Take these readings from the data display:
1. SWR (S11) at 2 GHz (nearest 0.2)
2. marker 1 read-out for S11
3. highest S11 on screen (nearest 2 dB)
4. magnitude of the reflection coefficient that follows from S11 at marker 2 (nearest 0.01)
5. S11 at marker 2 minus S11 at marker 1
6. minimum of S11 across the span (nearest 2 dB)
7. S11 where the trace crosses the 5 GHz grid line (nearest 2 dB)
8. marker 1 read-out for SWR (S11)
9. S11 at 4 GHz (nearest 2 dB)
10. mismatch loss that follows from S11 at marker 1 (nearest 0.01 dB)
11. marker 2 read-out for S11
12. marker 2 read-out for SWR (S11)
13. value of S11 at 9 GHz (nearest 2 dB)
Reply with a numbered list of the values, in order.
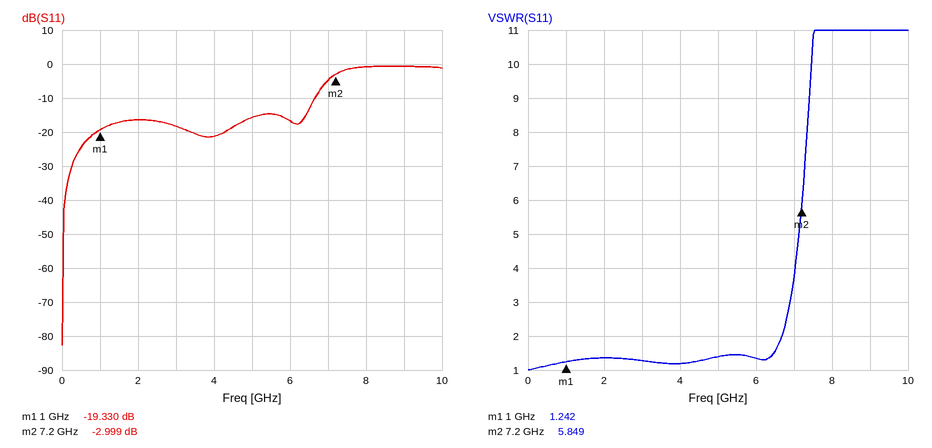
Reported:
1. 1.4
2. -19.330 dB
3. 0 dB
4. 0.71
5. 16.331 dB
6. -82 dB
7. -16 dB
8. 1.242
9. -22 dB
10. 0.05 dB
11. -2.999 dB
12. 5.849
13. 0 dB
